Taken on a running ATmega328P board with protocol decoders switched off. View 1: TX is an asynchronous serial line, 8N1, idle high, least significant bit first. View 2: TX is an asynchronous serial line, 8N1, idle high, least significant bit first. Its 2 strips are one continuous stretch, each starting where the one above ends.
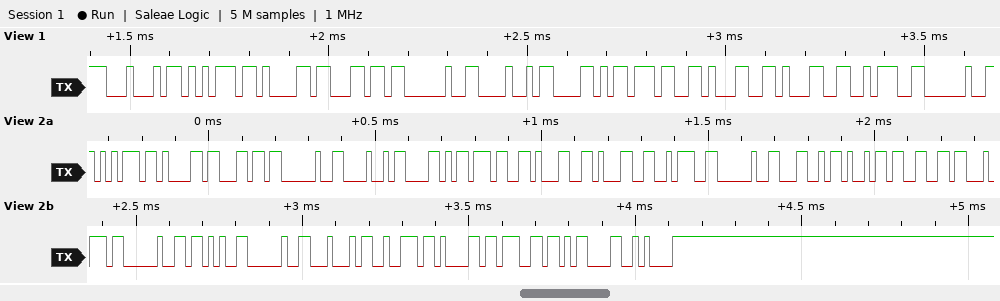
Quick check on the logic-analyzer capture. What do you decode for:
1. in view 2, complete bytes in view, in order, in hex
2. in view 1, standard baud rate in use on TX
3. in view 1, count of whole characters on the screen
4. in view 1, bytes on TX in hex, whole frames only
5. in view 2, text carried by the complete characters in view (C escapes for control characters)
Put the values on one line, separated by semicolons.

75 61 6C 20 48 58 37 31 31 3A 20 4C 69 66 74 20 2B 20 44 72 61 67 0D 0A; 57600 baud; 12; 44 75 61 6C 20 48 58 37 31 31 3A 20; "ual HX711: Lift + Drag\r\n"
